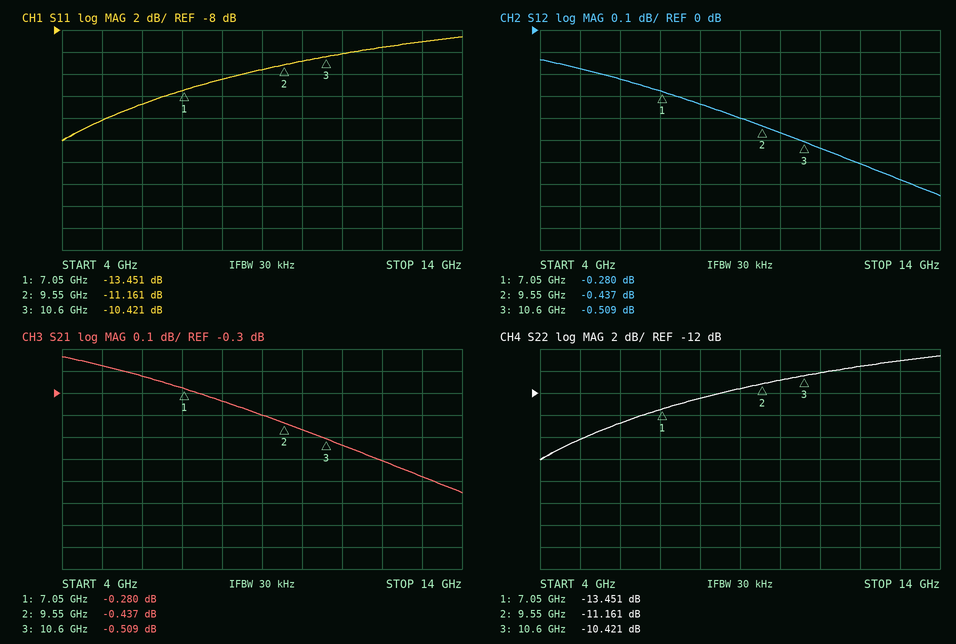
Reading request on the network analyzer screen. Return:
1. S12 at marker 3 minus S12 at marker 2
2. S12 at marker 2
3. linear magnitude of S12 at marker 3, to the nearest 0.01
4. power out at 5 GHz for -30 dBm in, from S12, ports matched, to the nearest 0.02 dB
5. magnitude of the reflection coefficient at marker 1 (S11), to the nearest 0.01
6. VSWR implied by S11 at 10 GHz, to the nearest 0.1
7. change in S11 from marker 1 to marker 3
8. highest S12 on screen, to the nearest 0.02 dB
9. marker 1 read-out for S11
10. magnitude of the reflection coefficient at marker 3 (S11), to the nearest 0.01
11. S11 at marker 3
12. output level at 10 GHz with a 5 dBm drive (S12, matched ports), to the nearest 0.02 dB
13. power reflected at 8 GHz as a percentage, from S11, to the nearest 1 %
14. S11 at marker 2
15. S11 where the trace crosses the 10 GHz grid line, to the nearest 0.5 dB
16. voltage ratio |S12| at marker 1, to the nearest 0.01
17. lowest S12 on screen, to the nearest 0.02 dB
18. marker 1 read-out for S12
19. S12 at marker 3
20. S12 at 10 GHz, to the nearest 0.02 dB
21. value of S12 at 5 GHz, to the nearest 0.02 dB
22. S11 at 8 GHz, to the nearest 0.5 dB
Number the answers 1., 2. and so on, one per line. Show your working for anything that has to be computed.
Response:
1. -0.509 − (-0.437) = -0.072 dB
2. -0.437 dB
3. 10^(-0.509/20) ≈ 0.94
4. -30 dBm + (-0.18 dB) = -30.18 dBm
5. 10^(-13.451/20) ≈ 0.21
6. |Γ| = 10^(-11/20) = 0.2818; VSWR = (1 + 0.2818)/(1 − 0.2818) ≈ 1.8
7. -10.421 − (-13.451) = 3.030 dB
8. -0.14 dB
9. -13.451 dB
10. 10^(-10.421/20) ≈ 0.30
11. -10.421 dB
12. 5 dBm + (-0.46 dB) = 4.54 dBm
13. 10^(-12.5/10) ≈ 6 %
14. -11.161 dB
15. -11.0 dB
16. 10^(-0.28/20) ≈ 0.97
17. -0.76 dB
18. -0.280 dB
19. -0.509 dB
20. -0.46 dB
21. -0.18 dB
22. -12.5 dB
